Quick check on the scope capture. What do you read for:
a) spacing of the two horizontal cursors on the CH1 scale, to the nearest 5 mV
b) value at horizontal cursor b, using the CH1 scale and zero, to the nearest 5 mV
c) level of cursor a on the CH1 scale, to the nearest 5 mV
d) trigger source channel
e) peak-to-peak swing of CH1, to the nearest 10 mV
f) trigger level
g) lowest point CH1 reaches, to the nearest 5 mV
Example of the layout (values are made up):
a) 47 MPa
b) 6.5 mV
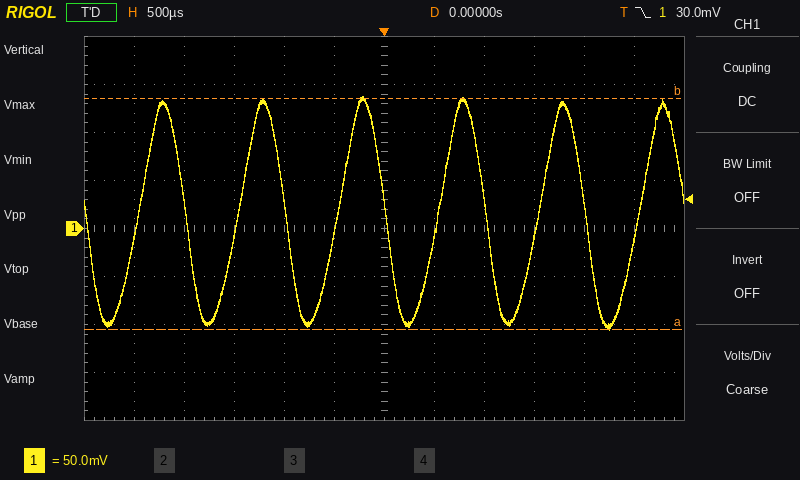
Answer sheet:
a) 240 mV
b) 135 mV
c) -105 mV
d) CH1
e) 240 mV
f) 30.0 mV
g) -105 mV
